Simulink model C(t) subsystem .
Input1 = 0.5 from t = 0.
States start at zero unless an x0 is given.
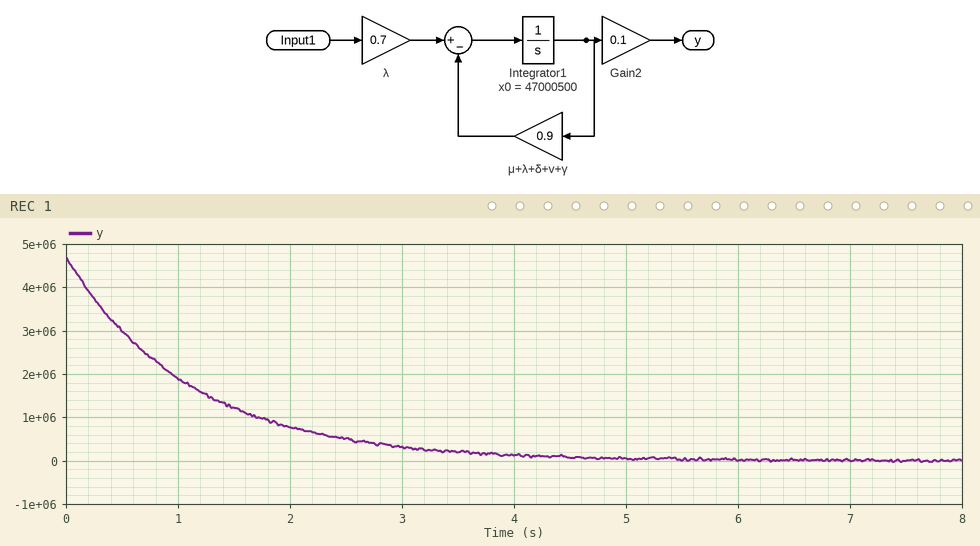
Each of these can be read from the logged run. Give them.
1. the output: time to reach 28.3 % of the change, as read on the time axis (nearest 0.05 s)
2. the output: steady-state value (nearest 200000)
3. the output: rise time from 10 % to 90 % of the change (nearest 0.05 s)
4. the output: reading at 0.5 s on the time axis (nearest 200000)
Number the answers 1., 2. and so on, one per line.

1. 0.35 s
2. 0
3. 2.45 s
4. 3000000
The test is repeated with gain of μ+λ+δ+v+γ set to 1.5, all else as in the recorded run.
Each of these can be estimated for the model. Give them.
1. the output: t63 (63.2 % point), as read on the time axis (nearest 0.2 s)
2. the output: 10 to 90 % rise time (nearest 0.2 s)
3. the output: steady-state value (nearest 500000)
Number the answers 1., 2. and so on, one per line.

1. 0.6 s
2. 1.4 s
3. 0
